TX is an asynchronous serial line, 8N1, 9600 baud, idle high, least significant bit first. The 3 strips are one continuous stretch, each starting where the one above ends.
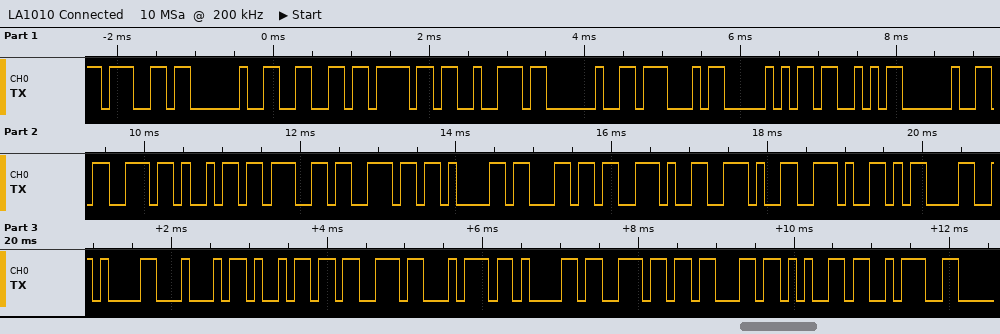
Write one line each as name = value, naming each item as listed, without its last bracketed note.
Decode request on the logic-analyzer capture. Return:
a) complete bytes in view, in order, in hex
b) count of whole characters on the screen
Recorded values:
complete bytes in view, in order, in hex = 67 20 66 6F 72 20 47 50 53 20 73 69 67 6E 61 6C 2E 2E 2E 0D 0A 44 69 73 74 61 6E 63 65 3A
count of whole characters on the screen = 30
